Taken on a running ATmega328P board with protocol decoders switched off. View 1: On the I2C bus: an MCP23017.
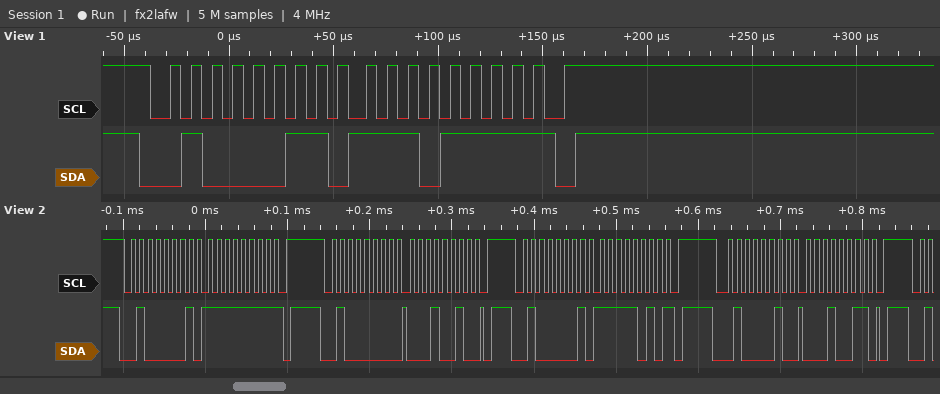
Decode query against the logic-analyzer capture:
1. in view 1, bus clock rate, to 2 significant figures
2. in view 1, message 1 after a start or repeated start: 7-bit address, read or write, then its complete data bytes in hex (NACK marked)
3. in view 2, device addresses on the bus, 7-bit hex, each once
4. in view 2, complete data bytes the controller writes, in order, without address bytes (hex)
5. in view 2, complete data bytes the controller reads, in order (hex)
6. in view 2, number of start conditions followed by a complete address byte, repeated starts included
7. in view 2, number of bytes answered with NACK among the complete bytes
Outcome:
100 kHz
0x21 read: EF NACK
0x20 0x21
12 13
FF FA
4
2
